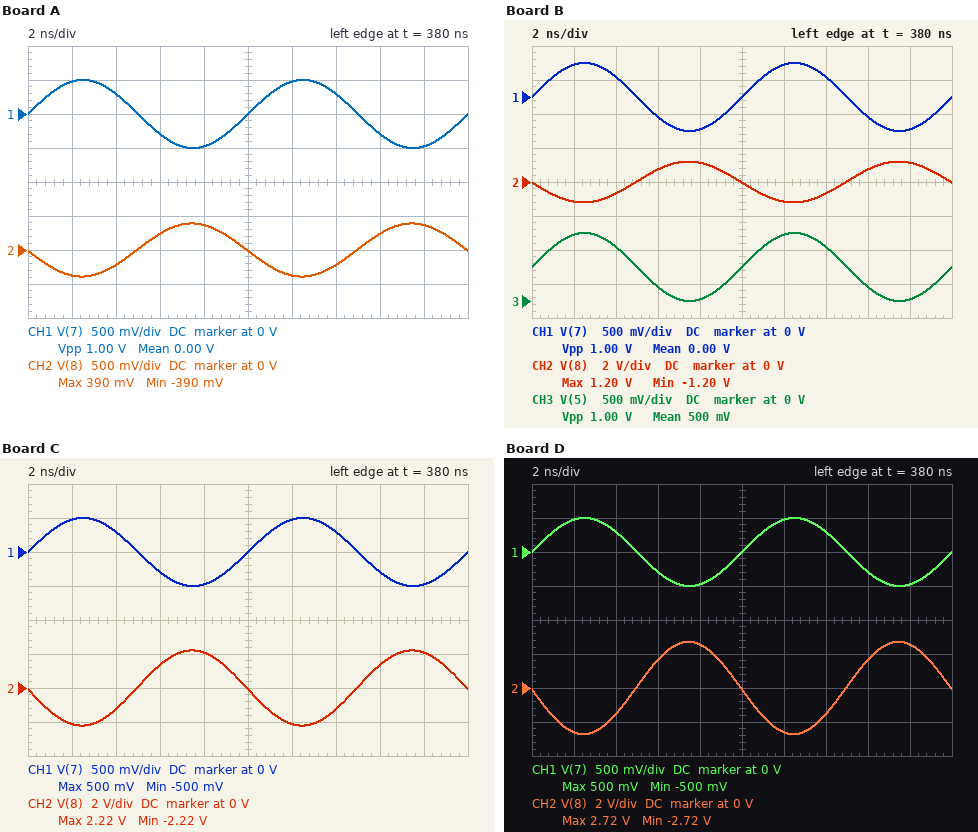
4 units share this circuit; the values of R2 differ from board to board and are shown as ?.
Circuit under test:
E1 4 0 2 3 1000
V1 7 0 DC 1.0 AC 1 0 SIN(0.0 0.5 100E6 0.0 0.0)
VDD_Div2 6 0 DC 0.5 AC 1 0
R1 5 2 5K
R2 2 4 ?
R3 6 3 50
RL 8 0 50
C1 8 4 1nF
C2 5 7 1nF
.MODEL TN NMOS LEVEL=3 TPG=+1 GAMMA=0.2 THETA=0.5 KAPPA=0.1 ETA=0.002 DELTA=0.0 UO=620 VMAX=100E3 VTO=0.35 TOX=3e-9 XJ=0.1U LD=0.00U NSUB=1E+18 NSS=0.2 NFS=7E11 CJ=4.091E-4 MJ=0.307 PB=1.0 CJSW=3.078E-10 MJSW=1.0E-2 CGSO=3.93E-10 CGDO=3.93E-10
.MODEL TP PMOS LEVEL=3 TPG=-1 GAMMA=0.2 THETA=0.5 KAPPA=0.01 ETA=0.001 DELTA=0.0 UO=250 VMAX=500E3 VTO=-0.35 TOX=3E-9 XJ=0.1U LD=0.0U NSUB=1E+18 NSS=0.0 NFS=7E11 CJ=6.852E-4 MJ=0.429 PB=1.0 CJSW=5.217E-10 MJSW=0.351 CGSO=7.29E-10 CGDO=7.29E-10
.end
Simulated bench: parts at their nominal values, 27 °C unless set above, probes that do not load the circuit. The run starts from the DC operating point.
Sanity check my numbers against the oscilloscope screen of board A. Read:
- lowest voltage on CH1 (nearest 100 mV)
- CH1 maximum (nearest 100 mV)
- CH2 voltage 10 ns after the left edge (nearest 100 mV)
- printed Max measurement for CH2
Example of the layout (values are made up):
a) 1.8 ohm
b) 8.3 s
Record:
a) -500 mV
b) 500 mV
c) 0 V
d) 390 mV
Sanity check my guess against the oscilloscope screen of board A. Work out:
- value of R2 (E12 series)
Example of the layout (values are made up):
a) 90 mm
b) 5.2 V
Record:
a) 3.9 kΩ
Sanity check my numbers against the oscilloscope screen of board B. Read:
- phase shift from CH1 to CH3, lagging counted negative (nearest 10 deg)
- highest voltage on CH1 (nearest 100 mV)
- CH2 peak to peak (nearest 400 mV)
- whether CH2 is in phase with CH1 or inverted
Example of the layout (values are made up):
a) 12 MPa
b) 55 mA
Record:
a) 0 deg
b) 500 mV
c) 2.4 V
d) inverted
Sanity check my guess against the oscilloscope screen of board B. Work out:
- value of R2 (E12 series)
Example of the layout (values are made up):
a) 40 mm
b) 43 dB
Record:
a) 12 kΩ
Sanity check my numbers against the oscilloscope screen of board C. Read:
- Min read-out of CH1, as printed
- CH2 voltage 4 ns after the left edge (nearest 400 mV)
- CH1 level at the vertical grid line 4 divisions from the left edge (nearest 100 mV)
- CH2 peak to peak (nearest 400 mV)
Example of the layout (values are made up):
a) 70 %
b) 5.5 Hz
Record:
a) -500 mV
b) -1.2 V
c) -500 mV
d) 4.4 V
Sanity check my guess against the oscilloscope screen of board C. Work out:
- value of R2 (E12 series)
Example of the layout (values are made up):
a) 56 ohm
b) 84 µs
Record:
a) 22 kΩ
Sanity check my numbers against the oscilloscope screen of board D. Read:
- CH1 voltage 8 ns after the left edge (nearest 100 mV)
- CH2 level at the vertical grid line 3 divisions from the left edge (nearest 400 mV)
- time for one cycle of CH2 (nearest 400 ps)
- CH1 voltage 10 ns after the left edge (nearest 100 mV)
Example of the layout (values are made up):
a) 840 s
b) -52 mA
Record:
a) -500 mV
b) 1.6 V
c) 10.0 ns
d) 0 V
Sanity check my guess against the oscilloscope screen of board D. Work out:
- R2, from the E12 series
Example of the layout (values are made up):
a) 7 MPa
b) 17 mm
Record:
a) 27 kΩ
